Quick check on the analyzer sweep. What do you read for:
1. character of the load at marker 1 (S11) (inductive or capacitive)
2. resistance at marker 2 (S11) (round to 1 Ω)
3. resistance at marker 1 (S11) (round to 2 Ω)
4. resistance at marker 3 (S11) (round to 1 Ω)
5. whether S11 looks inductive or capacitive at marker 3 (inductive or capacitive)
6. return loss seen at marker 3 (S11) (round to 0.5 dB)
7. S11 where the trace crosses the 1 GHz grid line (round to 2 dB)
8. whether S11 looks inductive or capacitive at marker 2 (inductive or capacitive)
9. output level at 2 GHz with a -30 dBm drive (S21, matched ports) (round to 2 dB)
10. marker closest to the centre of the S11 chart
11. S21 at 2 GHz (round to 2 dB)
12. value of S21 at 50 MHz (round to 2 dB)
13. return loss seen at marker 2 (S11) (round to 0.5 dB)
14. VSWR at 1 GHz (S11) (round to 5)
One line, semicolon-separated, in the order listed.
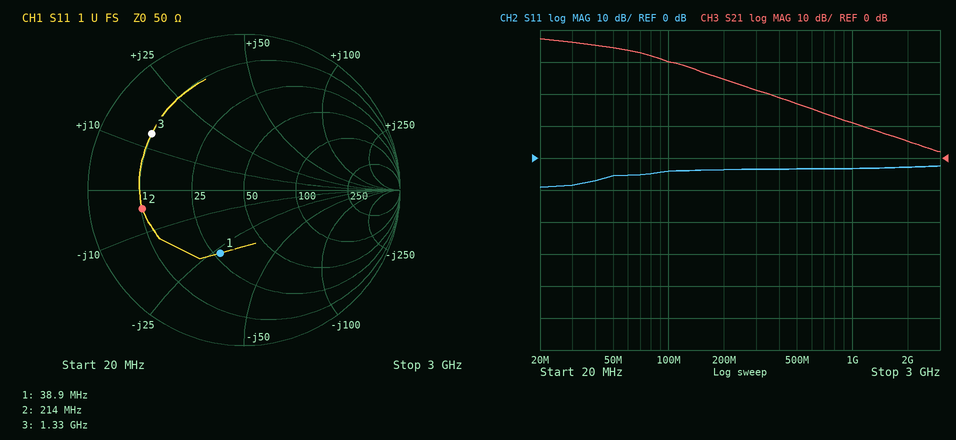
capacitive; 10 Ω; 28 Ω; 10 Ω; inductive; 3.0 dB; -4 dB; capacitive; -24 dBm; marker 1; 6 dB; 34 dB; 3.5 dB; 5
